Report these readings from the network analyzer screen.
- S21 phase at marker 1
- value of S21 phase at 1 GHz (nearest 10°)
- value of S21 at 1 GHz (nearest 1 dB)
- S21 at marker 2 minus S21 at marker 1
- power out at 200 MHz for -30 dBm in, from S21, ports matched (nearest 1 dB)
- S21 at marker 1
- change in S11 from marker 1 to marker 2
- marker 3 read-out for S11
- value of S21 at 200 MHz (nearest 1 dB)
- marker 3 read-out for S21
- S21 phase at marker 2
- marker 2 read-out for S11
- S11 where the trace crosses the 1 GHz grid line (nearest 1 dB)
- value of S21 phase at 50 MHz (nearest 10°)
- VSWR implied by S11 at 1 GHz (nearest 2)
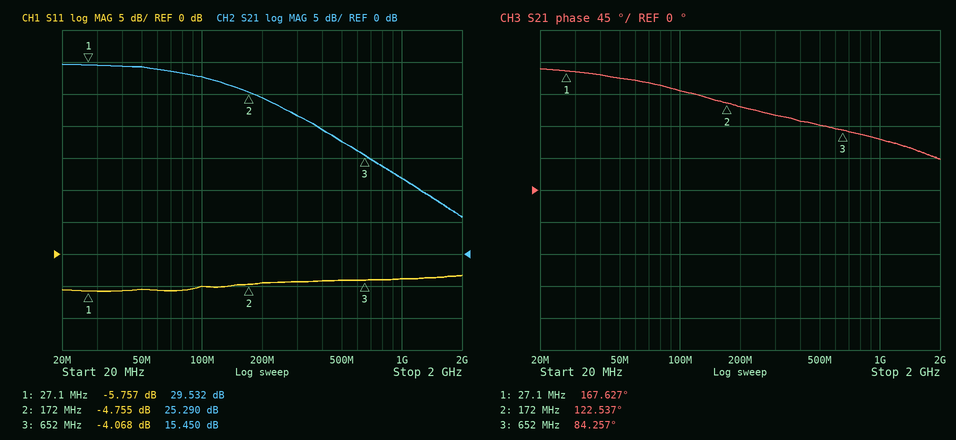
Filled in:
167.627°
70°
12 dB
-4.242 dB
-6 dBm
29.532 dB
1.002 dB
-4.068 dB
24 dB
15.450 dB
122.537°
-4.755 dB
-4 dB
160°
4
